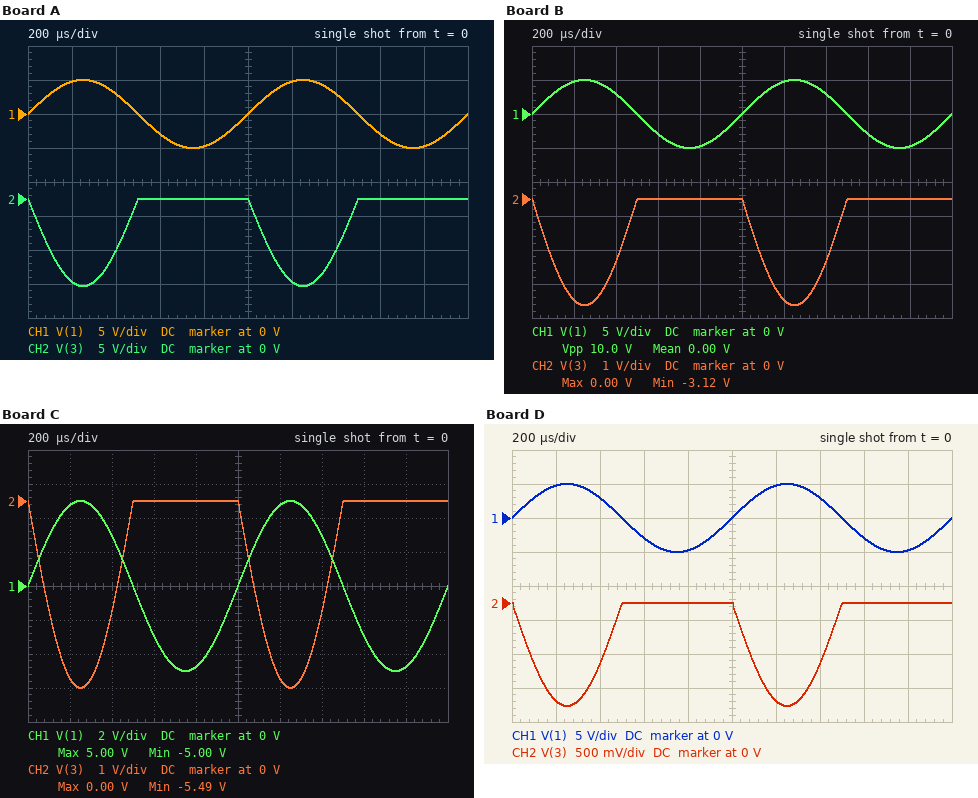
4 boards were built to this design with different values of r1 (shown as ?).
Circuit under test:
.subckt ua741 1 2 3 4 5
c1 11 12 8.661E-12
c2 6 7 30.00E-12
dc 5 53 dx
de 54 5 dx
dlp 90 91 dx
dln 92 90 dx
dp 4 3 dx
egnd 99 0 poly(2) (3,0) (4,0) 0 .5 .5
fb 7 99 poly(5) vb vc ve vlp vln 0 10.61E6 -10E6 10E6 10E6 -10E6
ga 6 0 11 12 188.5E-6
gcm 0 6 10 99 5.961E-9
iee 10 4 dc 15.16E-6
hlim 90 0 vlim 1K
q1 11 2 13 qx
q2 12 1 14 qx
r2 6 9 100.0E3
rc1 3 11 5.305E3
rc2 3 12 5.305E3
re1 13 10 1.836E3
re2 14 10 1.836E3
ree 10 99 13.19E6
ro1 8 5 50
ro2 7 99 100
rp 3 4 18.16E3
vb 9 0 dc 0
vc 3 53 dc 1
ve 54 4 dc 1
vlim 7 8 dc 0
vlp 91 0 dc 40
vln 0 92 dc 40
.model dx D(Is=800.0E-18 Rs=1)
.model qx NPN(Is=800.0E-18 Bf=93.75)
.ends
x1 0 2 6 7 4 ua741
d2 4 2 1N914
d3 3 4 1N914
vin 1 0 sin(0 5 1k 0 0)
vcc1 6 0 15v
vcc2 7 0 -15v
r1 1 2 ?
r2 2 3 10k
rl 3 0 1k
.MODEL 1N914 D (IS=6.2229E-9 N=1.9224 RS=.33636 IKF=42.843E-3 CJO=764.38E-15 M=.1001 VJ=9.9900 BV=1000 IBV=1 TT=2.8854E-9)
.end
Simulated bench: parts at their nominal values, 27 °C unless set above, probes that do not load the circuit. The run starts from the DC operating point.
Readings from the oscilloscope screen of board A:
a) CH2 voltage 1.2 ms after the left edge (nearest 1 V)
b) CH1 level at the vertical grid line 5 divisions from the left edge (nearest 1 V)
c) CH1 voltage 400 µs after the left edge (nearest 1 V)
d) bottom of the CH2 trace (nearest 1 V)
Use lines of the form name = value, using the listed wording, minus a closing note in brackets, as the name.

CH2 voltage 1.2 ms after the left edge = -12 V
CH1 level at the vertical grid line 5 divisions from the left edge = 0 V
CH1 voltage 400 µs after the left edge = 3 V
bottom of the CH2 trace = -13 V
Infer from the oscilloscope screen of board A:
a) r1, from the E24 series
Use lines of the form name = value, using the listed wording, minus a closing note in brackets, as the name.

r1, from the E24 series = 3.9 kΩ
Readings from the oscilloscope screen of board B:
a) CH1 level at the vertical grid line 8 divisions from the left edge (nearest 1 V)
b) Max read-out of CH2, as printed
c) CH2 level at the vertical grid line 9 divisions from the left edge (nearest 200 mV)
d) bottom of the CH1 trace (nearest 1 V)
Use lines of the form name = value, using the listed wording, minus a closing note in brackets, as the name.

CH1 level at the vertical grid line 8 divisions from the left edge = -3 V
Max read-out of CH2, as printed = 0.00 V
CH2 level at the vertical grid line 9 divisions from the left edge = 0 V
bottom of the CH1 trace = -5 V
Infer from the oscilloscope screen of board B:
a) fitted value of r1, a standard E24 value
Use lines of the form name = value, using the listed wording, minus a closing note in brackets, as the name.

fitted value of r1, a standard E24 value = 16 kΩ
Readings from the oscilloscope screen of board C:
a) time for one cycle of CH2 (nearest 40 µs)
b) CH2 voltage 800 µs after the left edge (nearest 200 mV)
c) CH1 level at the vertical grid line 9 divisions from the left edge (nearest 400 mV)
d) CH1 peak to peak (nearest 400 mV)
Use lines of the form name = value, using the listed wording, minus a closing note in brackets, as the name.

time for one cycle of CH2 = 1.00 ms
CH2 voltage 800 µs after the left edge = 0 V
CH1 level at the vertical grid line 9 divisions from the left edge = -4.8 V
CH1 peak to peak = 10.0 V
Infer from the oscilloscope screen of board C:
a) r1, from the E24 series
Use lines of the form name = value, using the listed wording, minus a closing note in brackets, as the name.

r1, from the E24 series = 9.1 kΩ
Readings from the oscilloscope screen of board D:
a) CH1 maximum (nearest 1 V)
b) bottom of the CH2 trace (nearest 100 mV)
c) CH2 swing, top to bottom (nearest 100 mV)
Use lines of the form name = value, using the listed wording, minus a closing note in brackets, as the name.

CH1 maximum = 5 V
bottom of the CH2 trace = -1.5 V
CH2 swing, top to bottom = 1.5 V
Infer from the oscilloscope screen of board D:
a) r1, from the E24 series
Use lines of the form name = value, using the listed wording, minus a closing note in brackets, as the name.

r1, from the E24 series = 33 kΩ
